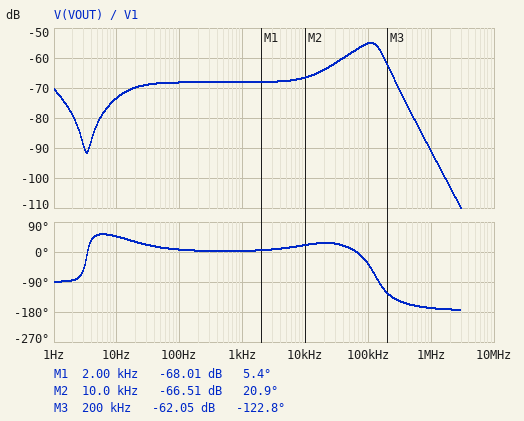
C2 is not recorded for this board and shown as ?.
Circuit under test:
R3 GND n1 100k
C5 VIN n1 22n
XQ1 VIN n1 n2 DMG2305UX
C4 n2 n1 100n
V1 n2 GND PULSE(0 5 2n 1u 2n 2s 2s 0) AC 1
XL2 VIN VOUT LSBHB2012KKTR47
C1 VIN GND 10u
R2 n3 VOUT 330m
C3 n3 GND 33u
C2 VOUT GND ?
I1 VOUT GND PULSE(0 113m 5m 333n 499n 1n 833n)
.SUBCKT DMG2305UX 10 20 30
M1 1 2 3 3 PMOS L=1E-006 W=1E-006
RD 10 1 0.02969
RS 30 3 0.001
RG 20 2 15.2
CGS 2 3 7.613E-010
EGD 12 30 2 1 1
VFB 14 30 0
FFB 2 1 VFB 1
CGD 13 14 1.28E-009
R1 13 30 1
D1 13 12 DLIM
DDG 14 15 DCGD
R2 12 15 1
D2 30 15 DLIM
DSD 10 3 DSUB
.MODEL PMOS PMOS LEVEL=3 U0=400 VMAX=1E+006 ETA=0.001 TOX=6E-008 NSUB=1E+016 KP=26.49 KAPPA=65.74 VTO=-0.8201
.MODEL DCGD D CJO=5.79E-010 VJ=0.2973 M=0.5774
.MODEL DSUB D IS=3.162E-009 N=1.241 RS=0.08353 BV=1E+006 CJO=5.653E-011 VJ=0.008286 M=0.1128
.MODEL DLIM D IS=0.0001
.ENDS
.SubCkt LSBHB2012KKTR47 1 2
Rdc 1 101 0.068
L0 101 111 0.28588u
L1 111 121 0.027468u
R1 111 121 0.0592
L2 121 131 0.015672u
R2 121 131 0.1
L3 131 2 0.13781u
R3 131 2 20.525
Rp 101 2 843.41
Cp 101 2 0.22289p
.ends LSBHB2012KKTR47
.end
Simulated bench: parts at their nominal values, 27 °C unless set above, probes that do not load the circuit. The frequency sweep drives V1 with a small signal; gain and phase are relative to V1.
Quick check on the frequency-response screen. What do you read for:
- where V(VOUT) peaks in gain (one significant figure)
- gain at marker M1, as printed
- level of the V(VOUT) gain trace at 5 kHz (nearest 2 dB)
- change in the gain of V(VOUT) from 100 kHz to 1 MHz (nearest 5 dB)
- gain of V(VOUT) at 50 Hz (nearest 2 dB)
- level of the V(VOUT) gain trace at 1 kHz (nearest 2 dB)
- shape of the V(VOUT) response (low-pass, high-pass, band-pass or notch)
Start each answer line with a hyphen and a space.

- 100 kHz
- -68.01 dB
- -68 dB
- -35 dB
- -68 dB
- -68 dB
- band-pass
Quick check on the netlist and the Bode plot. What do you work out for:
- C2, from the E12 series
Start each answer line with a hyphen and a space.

- 3.9 µF
